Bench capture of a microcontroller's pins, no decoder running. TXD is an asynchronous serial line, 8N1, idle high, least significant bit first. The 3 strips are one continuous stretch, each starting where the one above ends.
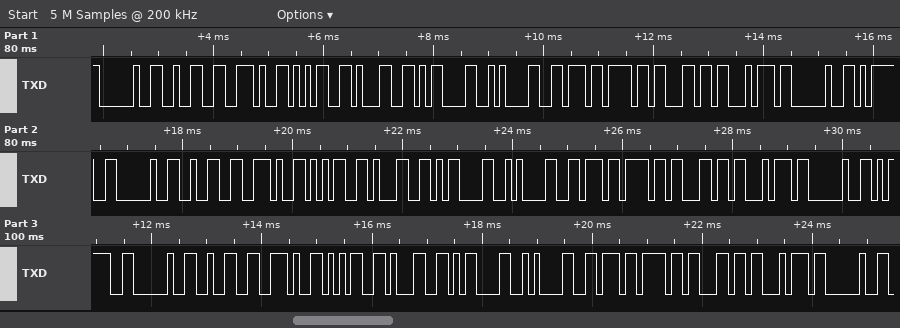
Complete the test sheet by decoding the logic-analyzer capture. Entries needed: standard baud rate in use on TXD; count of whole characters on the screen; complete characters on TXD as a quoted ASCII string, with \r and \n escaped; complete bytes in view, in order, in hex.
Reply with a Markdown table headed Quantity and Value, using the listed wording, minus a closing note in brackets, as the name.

| Quantity | Value |
|---|---|
| standard baud rate in use on TXD | 9600 baud |
| count of whole characters on the screen | 38 |
| complete characters on TXD as a quoted ASCII string, with \r and \n escaped | " 2.51\r\nvolt = 2.51\r\nvolt = 2.51\r\nvolt " |
| complete bytes in view, in order, in hex | 20 32 2E 35 31 0D 0A 76 6F 6C 74 20 3D 20 32 2E 35 31 0D 0A 76 6F 6C 74 20 3D 20 32 2E 35 31 0D 0A 76 6F 6C 74 20 |
